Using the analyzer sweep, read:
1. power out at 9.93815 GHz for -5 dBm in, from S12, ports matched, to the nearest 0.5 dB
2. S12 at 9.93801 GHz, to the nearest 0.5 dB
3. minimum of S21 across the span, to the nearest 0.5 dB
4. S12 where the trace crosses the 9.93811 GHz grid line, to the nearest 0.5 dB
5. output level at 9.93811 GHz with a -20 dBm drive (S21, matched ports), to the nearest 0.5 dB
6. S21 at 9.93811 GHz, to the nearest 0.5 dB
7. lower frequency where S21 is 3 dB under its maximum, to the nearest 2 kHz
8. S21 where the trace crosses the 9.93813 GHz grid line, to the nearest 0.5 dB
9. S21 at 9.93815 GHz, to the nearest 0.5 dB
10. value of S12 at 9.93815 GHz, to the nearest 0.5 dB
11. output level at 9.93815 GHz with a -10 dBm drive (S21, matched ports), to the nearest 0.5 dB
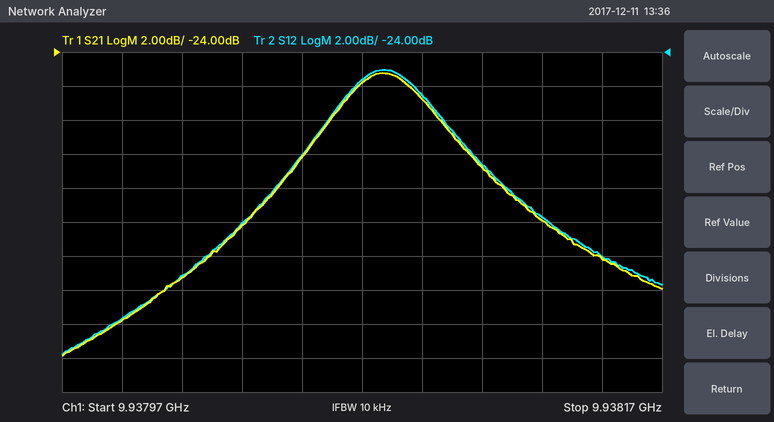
-41.0 dBm
-37.0 dB
-42.0 dB
-30.5 dB
-51.0 dBm
-31.0 dB
9.938058 GHz
-34.0 dB
-36.0 dB
-36.0 dB
-46.0 dBm
